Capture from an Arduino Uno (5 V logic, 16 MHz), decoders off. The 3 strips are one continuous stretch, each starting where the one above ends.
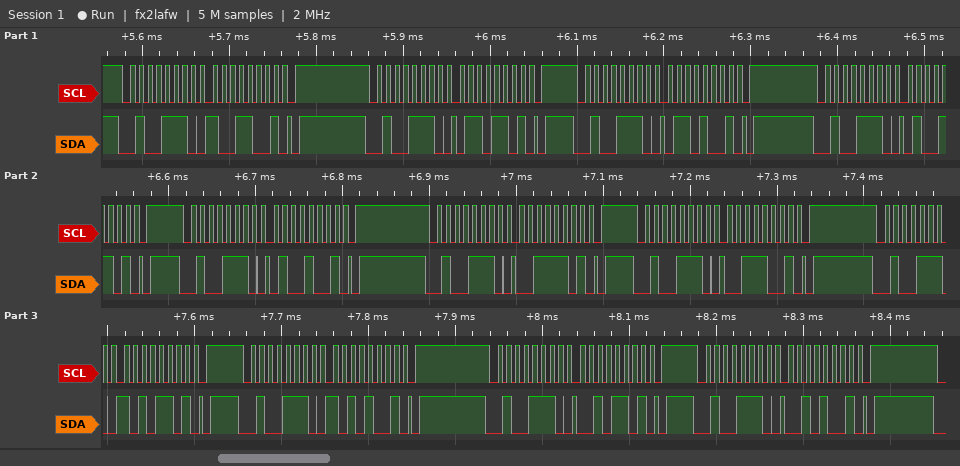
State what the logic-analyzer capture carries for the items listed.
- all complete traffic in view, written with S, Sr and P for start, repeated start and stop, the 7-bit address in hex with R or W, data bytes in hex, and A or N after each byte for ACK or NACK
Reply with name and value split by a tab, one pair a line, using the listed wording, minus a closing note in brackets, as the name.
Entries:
all complete traffic in view, written with S, Sr and P for start, repeated start and stop, the 7-bit address in hex with R or W, data bytes in hex, and A or N after each byte for ACK or NACK	S 27W A 99 A P S 27W A 6D A P S 27W A 69 A P S 27W A 4D A P S 27W A 49 A P S 27W A 3D A P S 27W A 39 A P S 27W A AD A P S 27W A A9 A P S 27W A 2D A P S 27W A 29 A P
